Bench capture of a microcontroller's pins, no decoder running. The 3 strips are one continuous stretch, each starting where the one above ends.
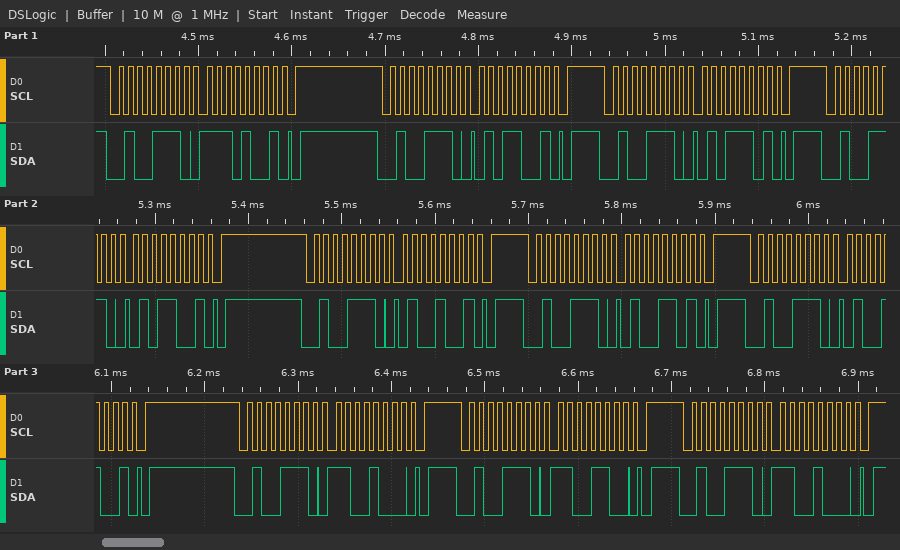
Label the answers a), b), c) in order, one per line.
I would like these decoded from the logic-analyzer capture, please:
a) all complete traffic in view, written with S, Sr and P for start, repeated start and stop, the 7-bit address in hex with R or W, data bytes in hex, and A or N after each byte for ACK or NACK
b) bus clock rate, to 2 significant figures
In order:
a) S 27W A E9 A P S 27W A 59 A P S 27W A 5D A P S 27W A 59 A P S 27W A 49 A P S 27W A 4D A P S 27W A 49 A P S 27W A C8 A P S 27W A CC A P S 27W A C8 A P
b) 100 kHz
